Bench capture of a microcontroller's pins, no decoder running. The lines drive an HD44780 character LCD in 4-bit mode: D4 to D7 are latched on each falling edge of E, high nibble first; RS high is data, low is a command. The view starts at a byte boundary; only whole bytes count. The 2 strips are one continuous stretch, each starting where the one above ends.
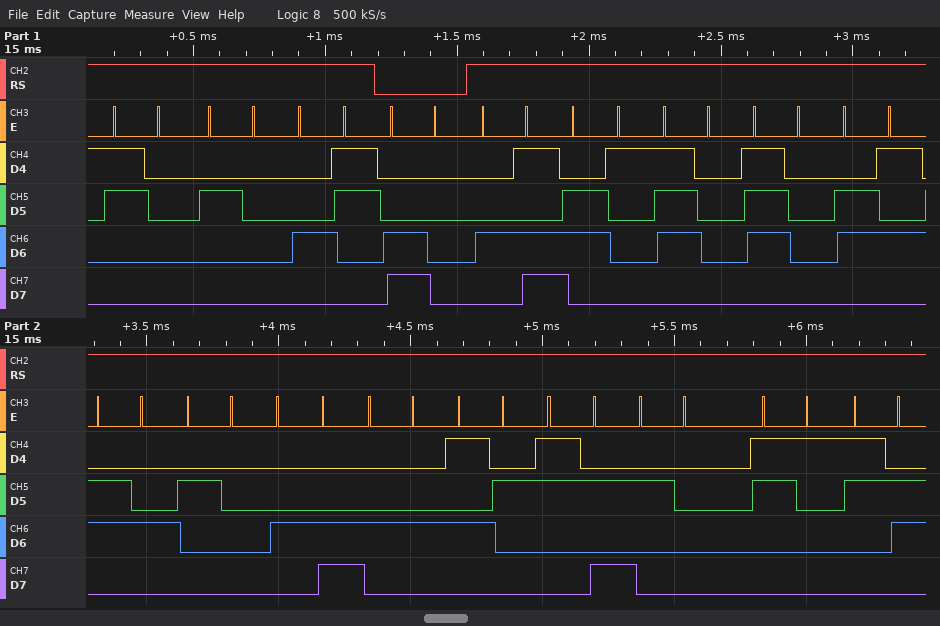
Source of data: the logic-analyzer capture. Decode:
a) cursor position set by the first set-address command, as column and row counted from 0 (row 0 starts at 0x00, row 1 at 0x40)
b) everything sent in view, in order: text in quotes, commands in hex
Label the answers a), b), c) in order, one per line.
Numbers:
a) column 0, row 1
b) "0 C" 0xC0 "Mapped LDR: 16"
